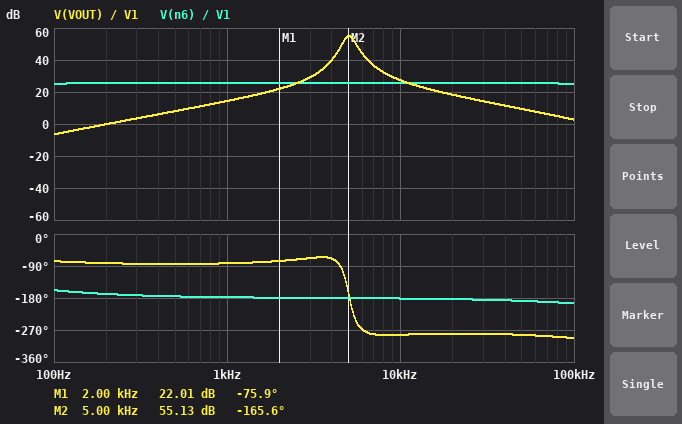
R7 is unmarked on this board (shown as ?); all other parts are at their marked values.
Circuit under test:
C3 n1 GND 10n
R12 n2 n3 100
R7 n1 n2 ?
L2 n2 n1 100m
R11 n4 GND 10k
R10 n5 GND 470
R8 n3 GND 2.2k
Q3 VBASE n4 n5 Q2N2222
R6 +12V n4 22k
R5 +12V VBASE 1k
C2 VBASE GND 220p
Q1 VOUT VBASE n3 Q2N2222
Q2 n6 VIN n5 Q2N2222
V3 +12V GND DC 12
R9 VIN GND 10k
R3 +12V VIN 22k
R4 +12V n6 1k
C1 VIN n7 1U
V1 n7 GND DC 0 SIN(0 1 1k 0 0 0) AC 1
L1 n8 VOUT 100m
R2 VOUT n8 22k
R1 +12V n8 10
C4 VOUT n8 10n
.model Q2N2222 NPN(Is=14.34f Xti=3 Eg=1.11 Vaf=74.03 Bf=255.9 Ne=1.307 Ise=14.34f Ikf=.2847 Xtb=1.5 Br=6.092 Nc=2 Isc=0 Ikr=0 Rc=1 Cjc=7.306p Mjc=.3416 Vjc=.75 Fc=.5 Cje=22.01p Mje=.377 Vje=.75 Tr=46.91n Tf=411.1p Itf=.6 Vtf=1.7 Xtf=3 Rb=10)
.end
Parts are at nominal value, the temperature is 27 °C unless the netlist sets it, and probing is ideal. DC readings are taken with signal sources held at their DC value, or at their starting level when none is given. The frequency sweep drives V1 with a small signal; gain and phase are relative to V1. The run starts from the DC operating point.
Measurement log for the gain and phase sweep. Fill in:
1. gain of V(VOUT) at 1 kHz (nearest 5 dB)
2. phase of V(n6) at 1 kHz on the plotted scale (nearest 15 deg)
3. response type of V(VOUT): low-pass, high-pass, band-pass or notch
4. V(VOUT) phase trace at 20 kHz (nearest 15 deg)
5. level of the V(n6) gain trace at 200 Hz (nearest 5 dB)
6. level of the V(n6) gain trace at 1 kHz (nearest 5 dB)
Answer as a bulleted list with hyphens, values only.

- 15 dB
- -180 deg
- band-pass
- -285 deg
- 25 dB
- 25 dB
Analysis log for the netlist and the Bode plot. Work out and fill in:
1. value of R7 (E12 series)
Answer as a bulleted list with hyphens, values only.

- 12 kΩ
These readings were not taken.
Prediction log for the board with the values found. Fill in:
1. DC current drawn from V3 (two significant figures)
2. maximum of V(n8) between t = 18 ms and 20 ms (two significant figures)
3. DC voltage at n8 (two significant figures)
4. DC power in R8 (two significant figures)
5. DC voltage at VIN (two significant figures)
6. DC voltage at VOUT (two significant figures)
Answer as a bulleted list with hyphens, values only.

- 11 mA
- 12 V
- 12 V
- 30 mW
- 3.6 V
- 12 V
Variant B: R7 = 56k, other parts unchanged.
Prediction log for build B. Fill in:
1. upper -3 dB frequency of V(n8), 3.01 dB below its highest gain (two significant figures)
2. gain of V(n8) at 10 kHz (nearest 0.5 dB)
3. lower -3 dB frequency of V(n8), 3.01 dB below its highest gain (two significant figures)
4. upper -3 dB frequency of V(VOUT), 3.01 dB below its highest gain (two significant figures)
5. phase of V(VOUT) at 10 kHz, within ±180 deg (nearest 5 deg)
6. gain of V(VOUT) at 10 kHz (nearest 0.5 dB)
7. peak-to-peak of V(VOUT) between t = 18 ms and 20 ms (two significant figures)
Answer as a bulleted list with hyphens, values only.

- 5.3 kHz
- -20.5 dB
- 4.8 kHz
- 5.2 kHz
- 70 deg
- 26.0 dB
- 19 V
